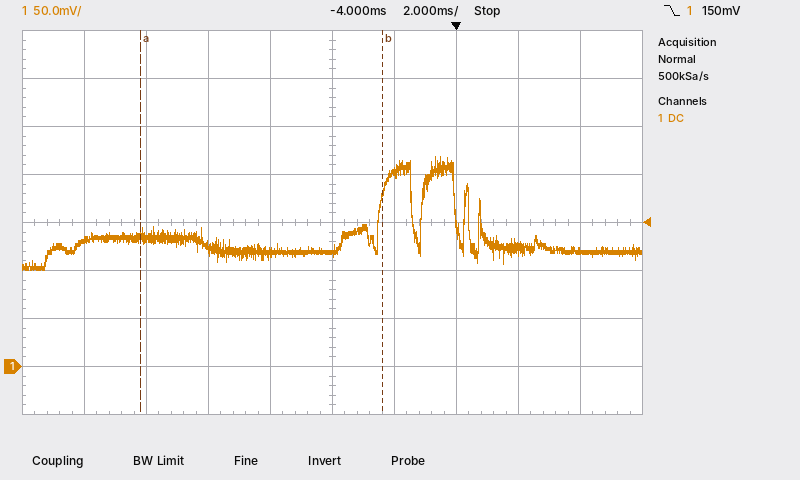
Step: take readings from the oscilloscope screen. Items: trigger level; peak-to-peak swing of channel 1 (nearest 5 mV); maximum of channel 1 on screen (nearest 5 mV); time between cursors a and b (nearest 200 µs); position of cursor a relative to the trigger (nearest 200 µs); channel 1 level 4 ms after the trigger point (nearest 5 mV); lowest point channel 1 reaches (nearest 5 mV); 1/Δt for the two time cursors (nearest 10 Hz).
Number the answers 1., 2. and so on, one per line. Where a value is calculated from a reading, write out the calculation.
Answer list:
1. 150 mV
2. 220 mV − (100 mV) = 120 mV
3. 220 mV
4. 7.8 ms
5. -10.2 ms
6. 120 mV
7. 100 mV
8. 1 / 7.8 ms ≈ 130 Hz
